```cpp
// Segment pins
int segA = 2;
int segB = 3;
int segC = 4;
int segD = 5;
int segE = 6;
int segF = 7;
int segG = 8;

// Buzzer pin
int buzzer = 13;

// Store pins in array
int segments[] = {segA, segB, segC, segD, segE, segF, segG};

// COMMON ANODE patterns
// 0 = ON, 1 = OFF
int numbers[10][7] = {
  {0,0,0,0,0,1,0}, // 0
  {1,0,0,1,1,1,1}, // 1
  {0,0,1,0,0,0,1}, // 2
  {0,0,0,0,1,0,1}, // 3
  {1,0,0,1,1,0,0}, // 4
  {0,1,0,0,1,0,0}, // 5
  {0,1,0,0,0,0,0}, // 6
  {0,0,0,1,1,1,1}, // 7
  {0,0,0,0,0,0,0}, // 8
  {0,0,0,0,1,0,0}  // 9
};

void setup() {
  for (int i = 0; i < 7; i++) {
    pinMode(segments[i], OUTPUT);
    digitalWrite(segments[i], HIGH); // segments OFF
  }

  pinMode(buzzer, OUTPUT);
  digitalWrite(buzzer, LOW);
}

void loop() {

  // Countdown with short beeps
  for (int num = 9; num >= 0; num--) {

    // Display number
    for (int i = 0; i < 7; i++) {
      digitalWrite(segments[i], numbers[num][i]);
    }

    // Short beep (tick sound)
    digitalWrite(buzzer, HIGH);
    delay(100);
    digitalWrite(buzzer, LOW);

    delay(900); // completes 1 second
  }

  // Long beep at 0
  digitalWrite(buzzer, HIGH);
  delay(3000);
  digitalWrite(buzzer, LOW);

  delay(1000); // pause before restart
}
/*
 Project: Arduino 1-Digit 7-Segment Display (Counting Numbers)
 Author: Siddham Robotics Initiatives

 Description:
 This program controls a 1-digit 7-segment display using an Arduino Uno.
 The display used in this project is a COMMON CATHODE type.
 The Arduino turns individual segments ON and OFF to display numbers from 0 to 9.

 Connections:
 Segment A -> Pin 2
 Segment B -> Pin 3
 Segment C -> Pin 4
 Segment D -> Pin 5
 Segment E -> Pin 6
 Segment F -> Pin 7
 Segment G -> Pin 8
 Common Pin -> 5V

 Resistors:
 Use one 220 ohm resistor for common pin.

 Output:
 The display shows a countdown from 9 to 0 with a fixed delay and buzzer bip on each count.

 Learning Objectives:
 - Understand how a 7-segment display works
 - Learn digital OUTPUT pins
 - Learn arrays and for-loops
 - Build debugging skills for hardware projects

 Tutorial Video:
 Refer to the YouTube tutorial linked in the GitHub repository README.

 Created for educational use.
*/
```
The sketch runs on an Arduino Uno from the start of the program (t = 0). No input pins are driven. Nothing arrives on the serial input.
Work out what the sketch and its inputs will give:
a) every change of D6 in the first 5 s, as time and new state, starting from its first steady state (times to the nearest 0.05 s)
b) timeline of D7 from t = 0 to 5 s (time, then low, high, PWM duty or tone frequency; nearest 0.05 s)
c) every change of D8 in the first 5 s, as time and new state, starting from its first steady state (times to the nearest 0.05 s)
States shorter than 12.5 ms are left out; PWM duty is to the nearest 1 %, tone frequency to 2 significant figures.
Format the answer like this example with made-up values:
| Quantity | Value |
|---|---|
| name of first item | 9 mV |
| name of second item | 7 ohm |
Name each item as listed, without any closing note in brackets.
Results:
| Quantity | Value |
|---|---|
| every change of D6 in the first 5 s, as time and new state, starting from its first steady state | 0 s high; 1 s low; 2 s high; 3 s low; 4 s high |
| timeline of D7 from t = 0 to 5 s | 0 s low; 2 s high; 3 s low |
| every change of D8 in the first 5 s, as time and new state, starting from its first steady state | 0 s low; 2 s high; 3 s low |
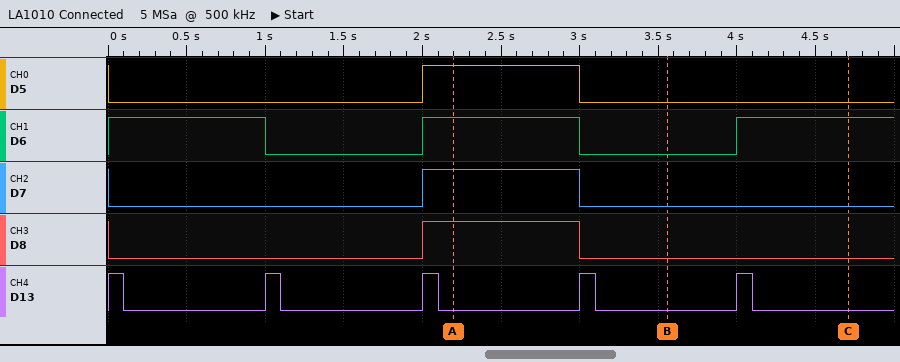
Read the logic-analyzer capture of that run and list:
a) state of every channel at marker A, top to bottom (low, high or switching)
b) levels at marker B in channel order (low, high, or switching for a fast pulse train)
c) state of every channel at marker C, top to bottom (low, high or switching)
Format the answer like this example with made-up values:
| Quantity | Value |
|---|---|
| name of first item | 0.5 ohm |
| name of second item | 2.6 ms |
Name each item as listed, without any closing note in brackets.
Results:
| Quantity | Value |
|---|---|
| state of every channel at marker A, top to bottom | D5 high, D6 high, D7 high, D8 high, D13 low |
| levels at marker B in channel order | D5 low, D6 low, D7 low, D8 low, D13 low |
| state of every channel at marker C, top to bottom | D5 low, D6 high, D7 low, D8 low, D13 low |
